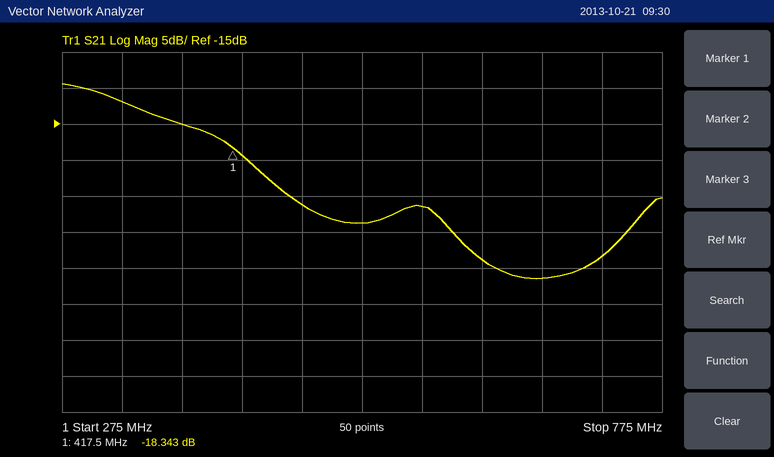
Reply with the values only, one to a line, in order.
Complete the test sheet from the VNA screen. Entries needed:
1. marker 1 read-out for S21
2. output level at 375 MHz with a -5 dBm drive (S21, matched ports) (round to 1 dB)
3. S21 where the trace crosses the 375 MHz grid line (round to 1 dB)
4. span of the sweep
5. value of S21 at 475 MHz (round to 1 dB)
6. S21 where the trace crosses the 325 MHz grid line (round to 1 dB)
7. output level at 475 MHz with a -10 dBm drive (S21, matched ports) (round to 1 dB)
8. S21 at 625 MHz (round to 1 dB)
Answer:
-18.343 dB
-20 dBm
-15 dB
500 MHz
-26 dB
-12 dB
-36 dBm
-34 dB
